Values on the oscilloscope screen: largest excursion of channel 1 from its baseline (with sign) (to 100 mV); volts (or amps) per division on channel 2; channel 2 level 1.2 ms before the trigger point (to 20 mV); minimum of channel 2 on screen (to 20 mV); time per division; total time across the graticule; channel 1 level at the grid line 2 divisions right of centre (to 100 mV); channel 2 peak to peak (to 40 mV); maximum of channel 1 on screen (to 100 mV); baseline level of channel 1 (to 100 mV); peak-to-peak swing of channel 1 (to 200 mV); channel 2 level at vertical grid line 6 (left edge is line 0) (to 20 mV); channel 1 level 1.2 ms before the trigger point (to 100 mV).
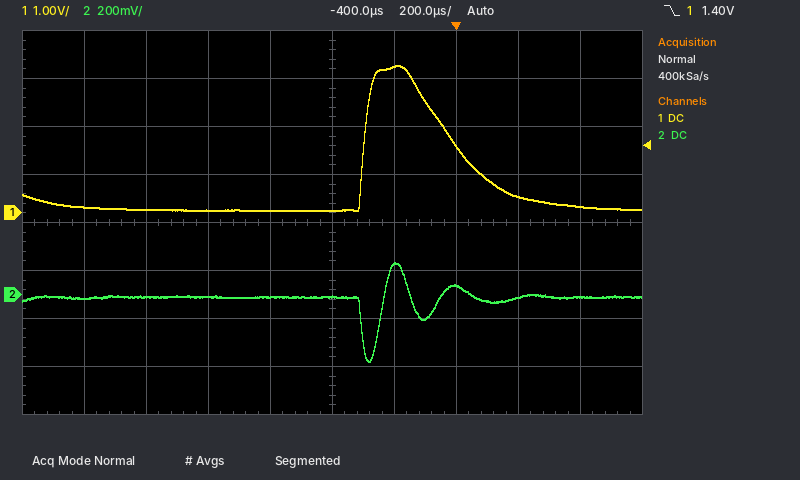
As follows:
+3.0 V
200 mV
-20 mV
-280 mV
200 µs
2 ms
1.4 V
400 mV
3.1 V
100 mV
3.0 V
120 mV
100 mV
